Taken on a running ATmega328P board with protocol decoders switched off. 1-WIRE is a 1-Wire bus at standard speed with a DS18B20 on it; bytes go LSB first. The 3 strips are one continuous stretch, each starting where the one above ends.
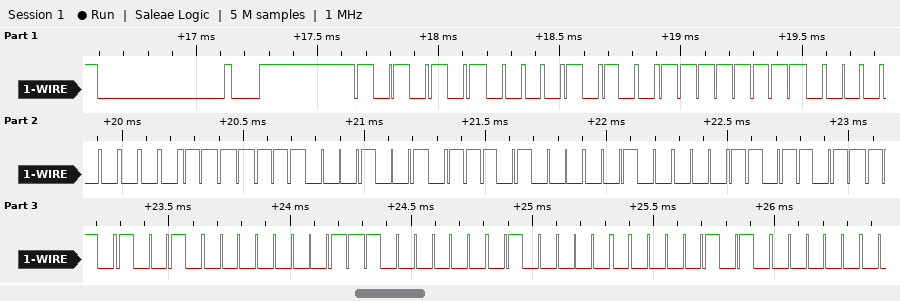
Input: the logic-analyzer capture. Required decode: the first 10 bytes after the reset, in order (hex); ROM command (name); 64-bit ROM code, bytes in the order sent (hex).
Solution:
55 28 FF 00 FE 48 17 04 DB 4B
Match ROM
28 FF 00 FE 48 17 04 DB
